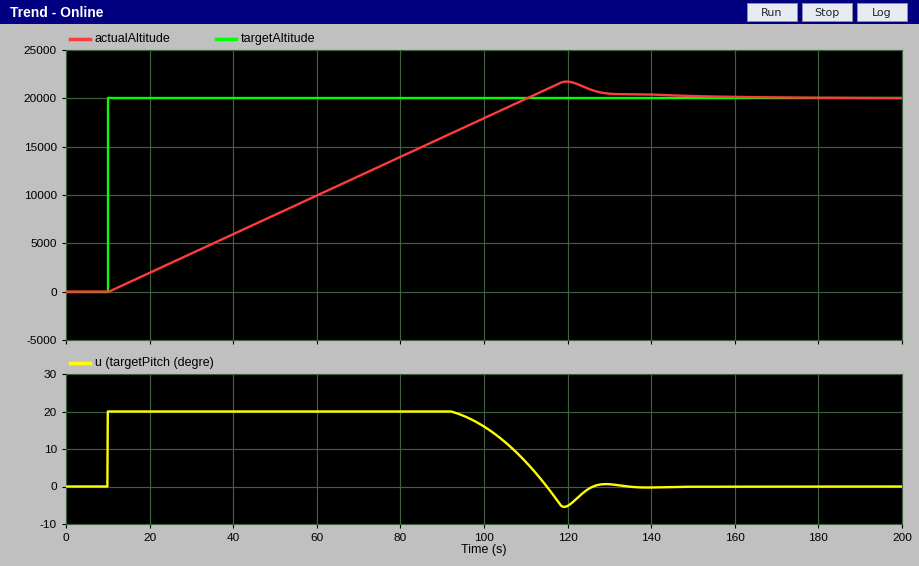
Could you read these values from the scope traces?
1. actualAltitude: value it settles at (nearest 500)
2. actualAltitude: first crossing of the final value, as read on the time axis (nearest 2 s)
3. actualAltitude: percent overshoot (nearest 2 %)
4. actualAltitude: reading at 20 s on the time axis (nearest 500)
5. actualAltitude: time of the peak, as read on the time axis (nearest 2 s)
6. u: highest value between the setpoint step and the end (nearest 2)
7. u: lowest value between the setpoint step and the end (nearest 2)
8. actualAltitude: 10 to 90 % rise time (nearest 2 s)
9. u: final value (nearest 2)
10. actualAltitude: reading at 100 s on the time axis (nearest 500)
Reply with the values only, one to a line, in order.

20000
110 s
8 %
2000
120 s
20
-6
80 s
0
18000
